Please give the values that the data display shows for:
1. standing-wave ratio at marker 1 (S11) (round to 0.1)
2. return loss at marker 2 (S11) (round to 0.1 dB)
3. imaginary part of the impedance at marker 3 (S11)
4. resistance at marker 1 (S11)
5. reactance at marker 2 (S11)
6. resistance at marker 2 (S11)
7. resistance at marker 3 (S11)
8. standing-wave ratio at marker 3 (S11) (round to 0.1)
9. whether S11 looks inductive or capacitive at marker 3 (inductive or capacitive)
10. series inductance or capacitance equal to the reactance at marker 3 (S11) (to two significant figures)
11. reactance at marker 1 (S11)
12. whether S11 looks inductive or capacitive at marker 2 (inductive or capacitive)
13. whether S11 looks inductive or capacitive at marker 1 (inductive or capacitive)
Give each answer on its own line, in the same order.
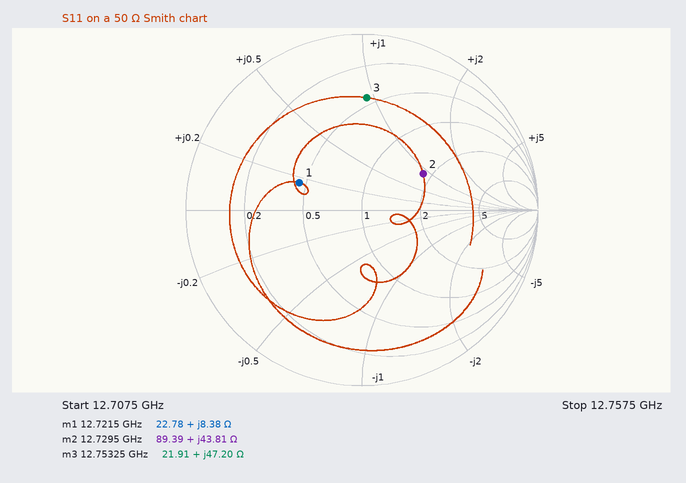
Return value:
2.3
7.9 dB
+47.20 Ω
22.78 Ω
+43.81 Ω
89.39 Ω
21.91 Ω
4.5
inductive
590 pH
+8.38 Ω
inductive
inductive
